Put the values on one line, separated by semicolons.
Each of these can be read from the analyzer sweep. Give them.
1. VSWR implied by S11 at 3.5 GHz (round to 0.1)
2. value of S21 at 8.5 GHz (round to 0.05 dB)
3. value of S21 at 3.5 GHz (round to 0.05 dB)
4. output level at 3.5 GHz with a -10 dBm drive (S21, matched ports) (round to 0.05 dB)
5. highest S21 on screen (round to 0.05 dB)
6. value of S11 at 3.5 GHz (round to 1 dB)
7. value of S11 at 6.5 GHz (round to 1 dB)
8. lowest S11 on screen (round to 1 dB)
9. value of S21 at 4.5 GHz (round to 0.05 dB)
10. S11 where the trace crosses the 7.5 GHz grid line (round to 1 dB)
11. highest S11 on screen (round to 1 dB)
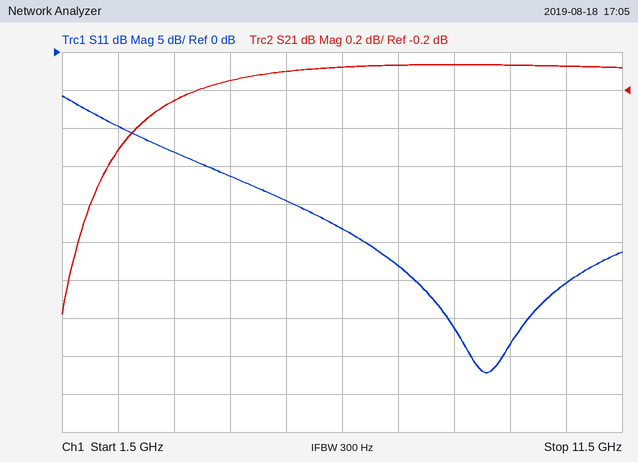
1.6; -0.05 dB; -0.25 dB; -10.25 dBm; -0.05 dB; -13 dB; -23 dB; -42 dB; -0.15 dB; -28 dB; -6 dB
